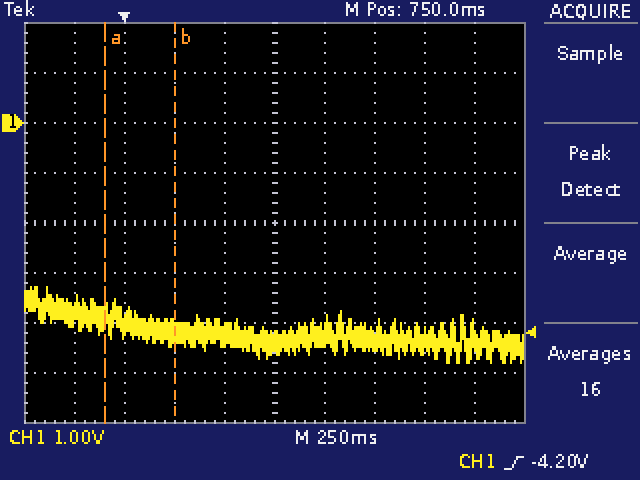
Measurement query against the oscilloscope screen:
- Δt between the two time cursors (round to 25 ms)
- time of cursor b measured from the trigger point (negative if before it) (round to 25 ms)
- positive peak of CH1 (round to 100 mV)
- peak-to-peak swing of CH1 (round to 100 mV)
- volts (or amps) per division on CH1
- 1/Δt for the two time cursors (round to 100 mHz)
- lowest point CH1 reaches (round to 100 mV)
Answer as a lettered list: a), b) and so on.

a) 350 ms
b) +250 ms
c) -3.3 V
d) 1.5 V
e) 1 V
f) 2.9 Hz
g) -4.8 V
